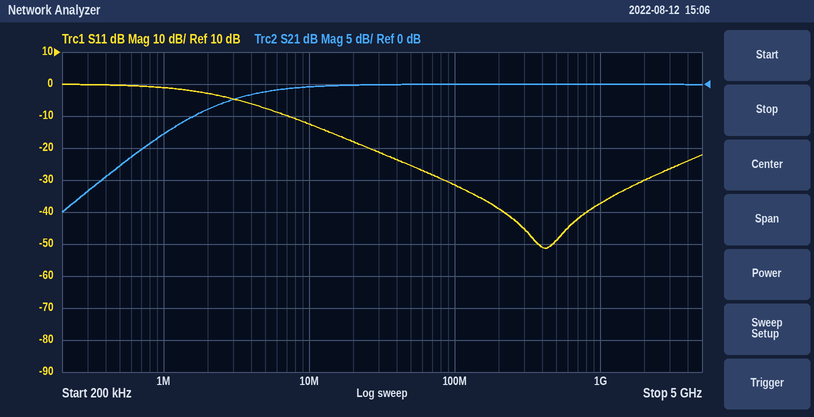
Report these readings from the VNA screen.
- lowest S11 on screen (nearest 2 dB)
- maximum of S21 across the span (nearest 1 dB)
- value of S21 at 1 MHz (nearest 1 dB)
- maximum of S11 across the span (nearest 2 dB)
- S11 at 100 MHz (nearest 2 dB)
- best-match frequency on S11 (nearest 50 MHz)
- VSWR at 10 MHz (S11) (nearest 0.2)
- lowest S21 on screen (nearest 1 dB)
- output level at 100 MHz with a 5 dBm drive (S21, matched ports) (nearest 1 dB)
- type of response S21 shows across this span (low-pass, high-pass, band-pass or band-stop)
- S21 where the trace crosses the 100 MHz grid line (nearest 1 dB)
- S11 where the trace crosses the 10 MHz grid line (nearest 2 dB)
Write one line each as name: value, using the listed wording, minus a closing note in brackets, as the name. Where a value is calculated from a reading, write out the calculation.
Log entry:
lowest S11 on screen: -52 dB
maximum of S21 across the span: 0 dB
value of S21 at 1 MHz: -8 dB
maximum of S11 across the span: 0 dB
S11 at 100 MHz: -32 dB
best-match frequency on S11: 400 MHz
VSWR at 10 MHz (S11): |Γ| = 10^(-12/20) = 0.2512; VSWR = (1 + 0.2512)/(1 − 0.2512) ≈ 1.67, so 1.6 to the nearest 0.2
lowest S21 on screen: -20 dB
output level at 100 MHz with a 5 dBm drive (S21, matched ports): 5 dBm + (0 dB) = 5 dBm
type of response S21 shows across this span: high-pass
S21 where the trace crosses the 100 MHz grid line: 0 dB
S11 where the trace crosses the 10 MHz grid line: -12 dB
